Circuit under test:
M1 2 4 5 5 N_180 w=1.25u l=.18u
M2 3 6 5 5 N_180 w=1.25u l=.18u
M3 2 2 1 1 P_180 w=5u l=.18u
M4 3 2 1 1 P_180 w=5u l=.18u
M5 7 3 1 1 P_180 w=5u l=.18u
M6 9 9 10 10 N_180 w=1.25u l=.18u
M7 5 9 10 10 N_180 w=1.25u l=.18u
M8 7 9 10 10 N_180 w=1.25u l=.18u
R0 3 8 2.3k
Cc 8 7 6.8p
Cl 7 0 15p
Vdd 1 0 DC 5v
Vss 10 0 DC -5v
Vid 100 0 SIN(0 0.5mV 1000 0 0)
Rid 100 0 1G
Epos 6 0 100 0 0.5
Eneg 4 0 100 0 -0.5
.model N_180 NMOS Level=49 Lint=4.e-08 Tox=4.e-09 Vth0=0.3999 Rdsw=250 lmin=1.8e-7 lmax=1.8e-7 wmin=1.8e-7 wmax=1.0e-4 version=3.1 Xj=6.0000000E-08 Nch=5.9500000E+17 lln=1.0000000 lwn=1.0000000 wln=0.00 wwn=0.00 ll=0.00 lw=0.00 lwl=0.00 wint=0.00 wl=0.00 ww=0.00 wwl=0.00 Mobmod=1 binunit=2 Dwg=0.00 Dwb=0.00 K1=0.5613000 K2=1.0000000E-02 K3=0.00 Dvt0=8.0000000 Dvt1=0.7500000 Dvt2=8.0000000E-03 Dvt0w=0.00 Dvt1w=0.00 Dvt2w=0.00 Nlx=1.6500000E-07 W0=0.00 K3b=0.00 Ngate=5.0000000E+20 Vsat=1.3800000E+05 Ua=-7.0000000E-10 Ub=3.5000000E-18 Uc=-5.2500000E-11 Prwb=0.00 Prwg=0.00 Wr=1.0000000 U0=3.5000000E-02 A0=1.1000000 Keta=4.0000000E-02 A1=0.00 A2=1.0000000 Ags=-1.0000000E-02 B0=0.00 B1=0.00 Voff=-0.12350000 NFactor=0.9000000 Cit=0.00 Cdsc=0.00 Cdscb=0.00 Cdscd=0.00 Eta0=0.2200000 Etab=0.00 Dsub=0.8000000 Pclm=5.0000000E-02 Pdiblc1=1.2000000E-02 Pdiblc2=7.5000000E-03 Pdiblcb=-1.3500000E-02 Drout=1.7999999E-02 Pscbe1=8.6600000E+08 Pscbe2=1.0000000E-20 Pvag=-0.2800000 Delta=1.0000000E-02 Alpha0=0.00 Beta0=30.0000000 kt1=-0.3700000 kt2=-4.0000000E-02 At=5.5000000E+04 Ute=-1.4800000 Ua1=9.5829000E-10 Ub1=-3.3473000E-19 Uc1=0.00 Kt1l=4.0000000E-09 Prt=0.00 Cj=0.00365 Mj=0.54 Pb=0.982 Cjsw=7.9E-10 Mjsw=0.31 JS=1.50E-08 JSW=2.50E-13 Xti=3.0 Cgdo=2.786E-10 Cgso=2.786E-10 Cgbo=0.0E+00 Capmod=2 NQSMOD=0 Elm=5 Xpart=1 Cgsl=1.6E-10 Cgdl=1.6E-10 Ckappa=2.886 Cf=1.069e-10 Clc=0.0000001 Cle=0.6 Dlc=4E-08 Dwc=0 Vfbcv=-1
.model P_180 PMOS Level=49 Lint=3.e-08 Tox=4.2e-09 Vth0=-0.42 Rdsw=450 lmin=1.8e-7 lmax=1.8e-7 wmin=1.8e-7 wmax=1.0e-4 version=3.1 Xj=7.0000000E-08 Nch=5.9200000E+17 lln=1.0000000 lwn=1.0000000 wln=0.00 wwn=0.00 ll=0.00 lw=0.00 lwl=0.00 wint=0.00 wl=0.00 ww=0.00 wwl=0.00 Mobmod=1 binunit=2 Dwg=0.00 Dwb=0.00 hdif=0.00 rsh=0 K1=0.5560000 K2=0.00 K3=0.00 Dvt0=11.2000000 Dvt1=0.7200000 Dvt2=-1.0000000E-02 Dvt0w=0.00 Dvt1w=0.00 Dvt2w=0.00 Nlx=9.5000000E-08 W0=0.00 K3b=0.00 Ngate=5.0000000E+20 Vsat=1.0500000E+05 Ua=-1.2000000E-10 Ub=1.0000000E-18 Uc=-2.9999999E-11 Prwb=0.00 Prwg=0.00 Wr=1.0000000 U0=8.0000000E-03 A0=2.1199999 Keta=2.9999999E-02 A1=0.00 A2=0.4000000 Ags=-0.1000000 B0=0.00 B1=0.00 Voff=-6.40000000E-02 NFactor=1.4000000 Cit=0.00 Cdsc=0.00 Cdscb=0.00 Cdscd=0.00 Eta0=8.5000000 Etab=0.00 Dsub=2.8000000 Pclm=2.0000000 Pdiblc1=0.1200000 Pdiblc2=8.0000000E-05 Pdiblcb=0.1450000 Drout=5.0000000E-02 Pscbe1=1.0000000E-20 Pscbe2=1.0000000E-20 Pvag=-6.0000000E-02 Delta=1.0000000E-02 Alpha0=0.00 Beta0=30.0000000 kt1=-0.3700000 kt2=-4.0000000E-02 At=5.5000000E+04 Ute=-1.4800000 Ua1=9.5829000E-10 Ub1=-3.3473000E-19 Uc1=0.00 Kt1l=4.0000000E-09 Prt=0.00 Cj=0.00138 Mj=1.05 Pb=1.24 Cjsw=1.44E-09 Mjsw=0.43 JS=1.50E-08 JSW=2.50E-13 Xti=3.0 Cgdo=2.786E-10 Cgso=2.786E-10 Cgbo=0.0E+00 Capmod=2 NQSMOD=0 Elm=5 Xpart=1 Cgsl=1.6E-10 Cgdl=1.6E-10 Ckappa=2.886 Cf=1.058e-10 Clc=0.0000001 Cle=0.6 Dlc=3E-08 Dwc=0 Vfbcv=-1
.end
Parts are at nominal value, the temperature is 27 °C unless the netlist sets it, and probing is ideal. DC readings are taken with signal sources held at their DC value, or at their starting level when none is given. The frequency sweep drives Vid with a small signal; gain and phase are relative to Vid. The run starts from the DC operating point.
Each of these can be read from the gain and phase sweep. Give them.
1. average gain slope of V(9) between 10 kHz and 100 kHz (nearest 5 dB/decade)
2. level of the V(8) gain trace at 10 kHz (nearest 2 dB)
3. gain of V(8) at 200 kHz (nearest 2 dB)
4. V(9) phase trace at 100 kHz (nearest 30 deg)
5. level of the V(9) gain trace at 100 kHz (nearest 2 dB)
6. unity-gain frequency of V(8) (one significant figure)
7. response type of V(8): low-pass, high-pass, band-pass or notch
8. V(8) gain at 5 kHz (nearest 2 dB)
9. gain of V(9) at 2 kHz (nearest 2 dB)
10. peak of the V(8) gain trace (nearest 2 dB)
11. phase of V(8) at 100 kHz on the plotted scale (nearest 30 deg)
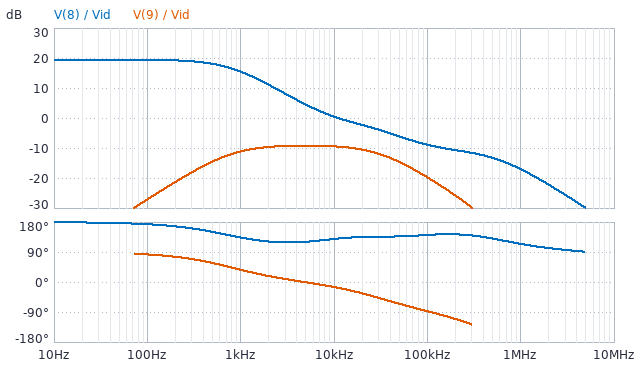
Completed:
-10 dB/decade
0 dB
-10 dB
-90 deg
-20 dB
10 kHz
low-pass
4 dB
-10 dB
20 dB
150 deg
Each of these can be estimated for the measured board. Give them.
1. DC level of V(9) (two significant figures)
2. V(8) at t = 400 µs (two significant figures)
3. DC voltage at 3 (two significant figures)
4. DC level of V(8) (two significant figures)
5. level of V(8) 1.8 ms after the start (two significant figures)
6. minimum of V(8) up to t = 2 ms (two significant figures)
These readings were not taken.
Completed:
-5.0 V
4.8 V
4.8 V
4.8 V
4.8 V
4.8 V
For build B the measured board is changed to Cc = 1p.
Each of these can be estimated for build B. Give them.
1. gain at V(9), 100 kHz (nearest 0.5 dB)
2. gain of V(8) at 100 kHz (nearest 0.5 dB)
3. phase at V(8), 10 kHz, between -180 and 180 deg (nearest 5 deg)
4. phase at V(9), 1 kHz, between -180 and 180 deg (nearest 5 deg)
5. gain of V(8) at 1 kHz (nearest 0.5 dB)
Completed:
-4.0 dB
5.0 dB
145 deg
75 deg
19.5 dB
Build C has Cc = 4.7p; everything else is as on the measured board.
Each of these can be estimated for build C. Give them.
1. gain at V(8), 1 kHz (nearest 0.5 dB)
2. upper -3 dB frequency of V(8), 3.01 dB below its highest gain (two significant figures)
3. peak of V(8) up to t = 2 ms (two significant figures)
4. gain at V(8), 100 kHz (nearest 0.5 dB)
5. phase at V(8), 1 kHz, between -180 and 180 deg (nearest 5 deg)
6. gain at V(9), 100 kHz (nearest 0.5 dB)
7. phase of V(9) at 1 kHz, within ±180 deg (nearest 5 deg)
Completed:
17.0 dB
1.2 kHz
4.8 V
-6.5 dB
145 deg
-16.5 dB
45 deg
